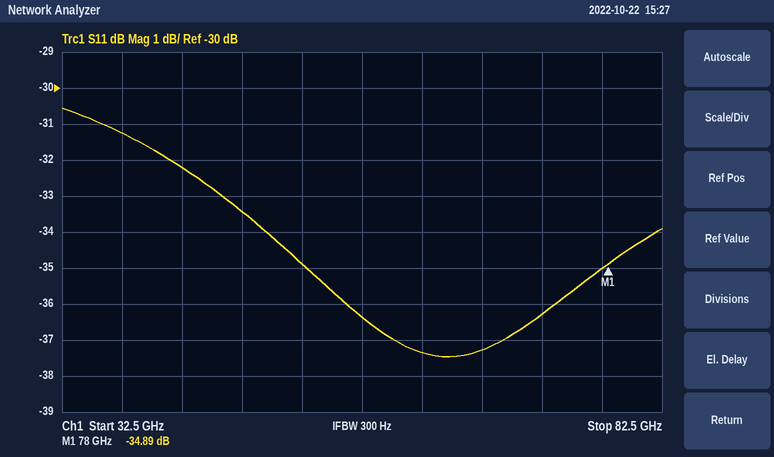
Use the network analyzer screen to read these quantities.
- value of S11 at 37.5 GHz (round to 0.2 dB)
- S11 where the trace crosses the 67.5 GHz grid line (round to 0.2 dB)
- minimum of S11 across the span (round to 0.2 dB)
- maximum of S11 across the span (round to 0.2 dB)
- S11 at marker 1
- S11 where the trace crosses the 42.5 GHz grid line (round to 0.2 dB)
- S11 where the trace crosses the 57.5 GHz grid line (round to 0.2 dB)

-31.2 dB
-37.2 dB
-37.4 dB
-30.6 dB
-34.89 dB
-32.2 dB
-36.4 dB
